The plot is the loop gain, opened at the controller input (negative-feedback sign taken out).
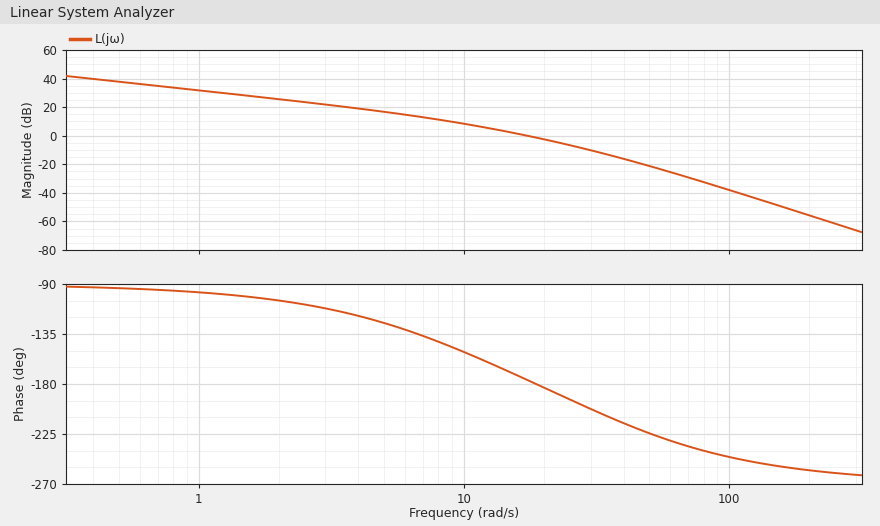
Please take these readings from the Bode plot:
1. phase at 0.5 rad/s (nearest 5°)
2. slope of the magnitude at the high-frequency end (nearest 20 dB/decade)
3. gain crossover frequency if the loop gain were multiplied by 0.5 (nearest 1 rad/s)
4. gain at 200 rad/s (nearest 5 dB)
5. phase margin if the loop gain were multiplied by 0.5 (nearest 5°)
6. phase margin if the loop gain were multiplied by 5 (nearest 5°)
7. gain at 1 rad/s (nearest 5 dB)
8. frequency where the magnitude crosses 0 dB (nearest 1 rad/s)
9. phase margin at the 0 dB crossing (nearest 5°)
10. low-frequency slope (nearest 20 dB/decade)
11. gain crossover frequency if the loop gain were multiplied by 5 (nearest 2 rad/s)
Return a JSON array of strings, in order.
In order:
["-95°", "-60 dB/decade", "12 rad/s", "-55 dB", "20°", "-30°", "30 dB", "17 rad/s", "5°", "-20 dB/decade", "36 rad/s"]
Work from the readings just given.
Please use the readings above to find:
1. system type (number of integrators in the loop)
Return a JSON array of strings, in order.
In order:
["1"]
